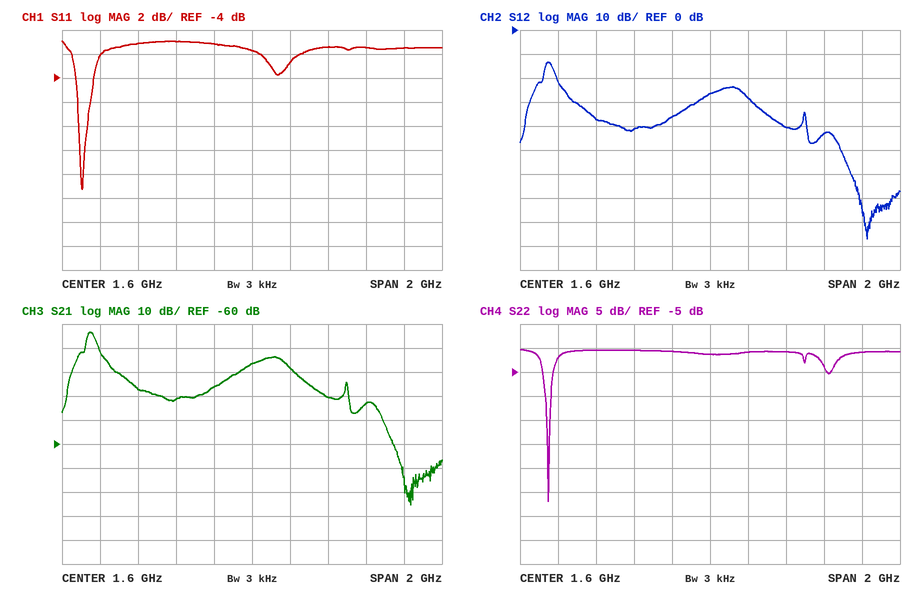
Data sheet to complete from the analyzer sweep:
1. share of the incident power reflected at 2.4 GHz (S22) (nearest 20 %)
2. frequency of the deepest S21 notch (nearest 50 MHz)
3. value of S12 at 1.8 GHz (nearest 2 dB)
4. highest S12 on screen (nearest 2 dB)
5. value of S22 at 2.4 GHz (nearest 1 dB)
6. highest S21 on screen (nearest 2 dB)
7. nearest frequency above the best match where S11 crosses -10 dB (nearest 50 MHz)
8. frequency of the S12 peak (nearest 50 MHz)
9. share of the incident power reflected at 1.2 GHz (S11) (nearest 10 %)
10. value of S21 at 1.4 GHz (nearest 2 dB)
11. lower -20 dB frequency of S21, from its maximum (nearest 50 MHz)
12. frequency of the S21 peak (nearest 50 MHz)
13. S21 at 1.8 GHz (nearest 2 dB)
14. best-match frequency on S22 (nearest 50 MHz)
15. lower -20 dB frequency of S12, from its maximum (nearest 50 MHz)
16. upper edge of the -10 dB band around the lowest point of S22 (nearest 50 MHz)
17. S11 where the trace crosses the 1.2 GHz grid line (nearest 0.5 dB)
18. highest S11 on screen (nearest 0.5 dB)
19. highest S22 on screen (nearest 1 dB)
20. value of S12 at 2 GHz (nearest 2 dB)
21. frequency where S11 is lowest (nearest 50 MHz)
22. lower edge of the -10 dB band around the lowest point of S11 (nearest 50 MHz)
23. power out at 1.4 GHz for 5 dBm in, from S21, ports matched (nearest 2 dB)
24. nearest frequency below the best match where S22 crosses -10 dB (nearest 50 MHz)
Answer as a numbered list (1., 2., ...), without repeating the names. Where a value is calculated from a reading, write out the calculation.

1. 10^(-1/10) ≈ 79.4 %, so 80 % to the nearest 20 %
2. 2.45 GHz
3. -28 dB
4. -14 dB
5. -1 dB
6. -14 dB
7. 700 MHz
8. 750 MHz
9. 10^(-1/10) ≈ 79.4 %, so 80 % to the nearest 10 %
10. -36 dB
11. 650 MHz
12. 750 MHz
13. -28 dB
14. 750 MHz
15. 650 MHz
16. 750 MHz
17. -1.0 dB
18. -1.0 dB
19. 0 dB
20. -40 dB
21. 700 MHz
22. 700 MHz
23. 5 dBm + (-36 dB) = -32 dBm
24. 750 MHz
